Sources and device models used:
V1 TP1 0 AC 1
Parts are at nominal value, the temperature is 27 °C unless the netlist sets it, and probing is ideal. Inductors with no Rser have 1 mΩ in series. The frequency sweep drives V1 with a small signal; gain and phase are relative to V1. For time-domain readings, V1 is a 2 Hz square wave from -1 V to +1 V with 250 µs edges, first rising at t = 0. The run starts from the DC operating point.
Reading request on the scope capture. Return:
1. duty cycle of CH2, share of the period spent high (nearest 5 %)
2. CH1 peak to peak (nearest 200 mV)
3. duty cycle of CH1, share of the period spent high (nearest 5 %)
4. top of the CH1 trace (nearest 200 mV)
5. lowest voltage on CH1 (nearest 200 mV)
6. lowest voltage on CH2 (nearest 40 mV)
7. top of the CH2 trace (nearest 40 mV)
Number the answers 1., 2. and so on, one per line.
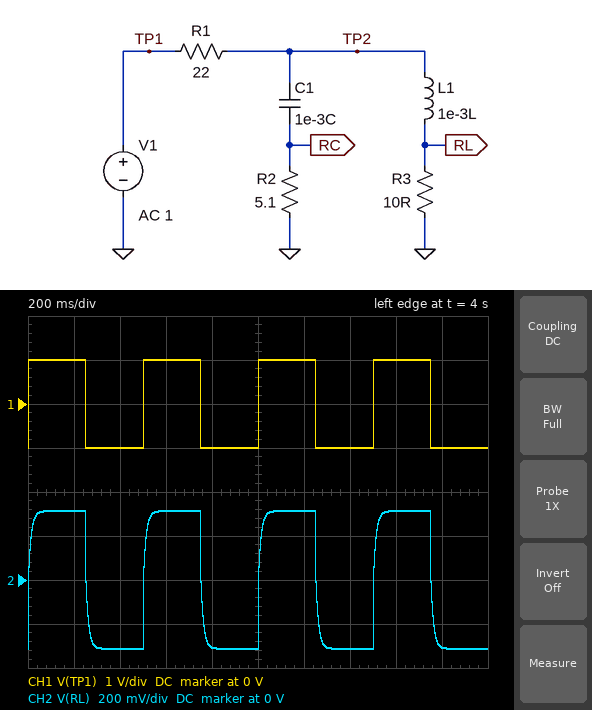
1. 50 %
2. 2.0 V
3. 50 %
4. 1.0 V
5. -1.0 V
6. -320 mV
7. 320 mV
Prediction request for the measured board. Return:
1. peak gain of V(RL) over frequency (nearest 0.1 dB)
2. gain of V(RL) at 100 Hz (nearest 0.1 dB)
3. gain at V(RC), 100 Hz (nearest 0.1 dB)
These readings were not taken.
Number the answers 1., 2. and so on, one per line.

1. -10.1 dB
2. -17.2 dB
3. -17.6 dB
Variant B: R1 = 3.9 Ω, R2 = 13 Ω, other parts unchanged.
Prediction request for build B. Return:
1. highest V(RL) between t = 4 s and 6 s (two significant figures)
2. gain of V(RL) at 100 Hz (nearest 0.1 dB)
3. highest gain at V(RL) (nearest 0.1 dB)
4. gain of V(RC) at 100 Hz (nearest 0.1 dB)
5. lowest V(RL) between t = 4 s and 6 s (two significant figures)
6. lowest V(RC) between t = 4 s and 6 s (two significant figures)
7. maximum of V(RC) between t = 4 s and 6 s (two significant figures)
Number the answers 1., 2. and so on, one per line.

1. 720 mV
2. -4.5 dB
3. -2.9 dB
4. -4.6 dB
5. -720 mV
6. -1.2 V
7. 1.2 V
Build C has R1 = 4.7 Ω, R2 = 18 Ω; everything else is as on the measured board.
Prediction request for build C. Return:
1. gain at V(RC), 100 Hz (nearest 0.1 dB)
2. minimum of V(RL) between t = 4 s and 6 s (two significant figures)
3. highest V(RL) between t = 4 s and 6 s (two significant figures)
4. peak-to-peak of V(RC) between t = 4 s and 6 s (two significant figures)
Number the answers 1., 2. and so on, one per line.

1. -4.8 dB
2. -680 mV
3. 680 mV
4. 2.3 V
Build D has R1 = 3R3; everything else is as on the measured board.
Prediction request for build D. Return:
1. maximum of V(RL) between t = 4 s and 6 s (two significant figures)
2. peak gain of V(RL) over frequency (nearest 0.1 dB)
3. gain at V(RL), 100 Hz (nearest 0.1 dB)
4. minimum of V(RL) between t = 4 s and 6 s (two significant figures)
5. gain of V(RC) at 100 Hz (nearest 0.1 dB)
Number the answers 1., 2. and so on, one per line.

1. 750 mV
2. -2.5 dB
3. -5.7 dB
4. -750 mV
5. -6.1 dB
